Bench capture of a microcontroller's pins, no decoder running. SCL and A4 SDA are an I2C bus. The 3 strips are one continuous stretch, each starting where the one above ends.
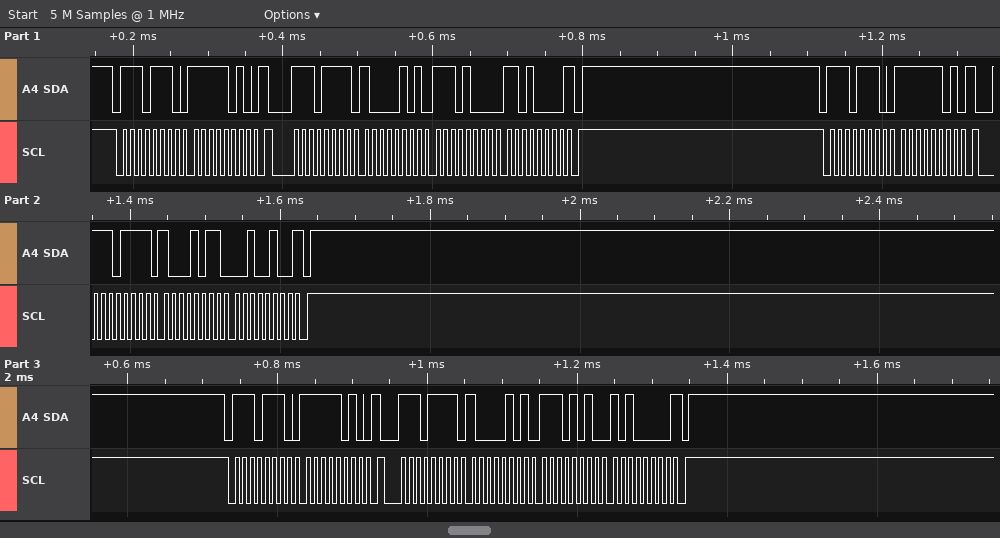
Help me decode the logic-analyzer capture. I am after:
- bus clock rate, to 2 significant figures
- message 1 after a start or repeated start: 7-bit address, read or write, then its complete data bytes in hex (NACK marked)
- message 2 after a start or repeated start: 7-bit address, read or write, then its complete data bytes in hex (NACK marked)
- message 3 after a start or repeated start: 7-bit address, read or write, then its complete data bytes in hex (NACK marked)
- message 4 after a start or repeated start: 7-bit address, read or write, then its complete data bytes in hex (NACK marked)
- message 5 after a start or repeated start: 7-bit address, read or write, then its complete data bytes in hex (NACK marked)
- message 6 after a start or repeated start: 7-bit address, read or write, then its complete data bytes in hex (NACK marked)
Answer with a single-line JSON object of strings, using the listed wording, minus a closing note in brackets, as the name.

{"bus clock rate, to 2 significant figures": "100 kHz", "message 1 after a start or repeated start: 7-bit address, read or write, then its complete data bytes in hex": "0x77 write: FA", "message 2 after a start or repeated start: 7-bit address, read or write, then its complete data bytes in hex": "0x77 read: 85 E8 D0 NACK", "message 3 after a start or repeated start: 7-bit address, read or write, then its complete data bytes in hex": "0x77 write: FD", "message 4 after a start or repeated start: 7-bit address, read or write, then its complete data bytes in hex": "0x77 read: 8B 24 NACK", "message 5 after a start or repeated start: 7-bit address, read or write, then its complete data bytes in hex": "0x77 write: FA", "message 6 after a start or repeated start: 7-bit address, read or write, then its complete data bytes in hex": "0x77 read: 85 EA A0 NACK"}
